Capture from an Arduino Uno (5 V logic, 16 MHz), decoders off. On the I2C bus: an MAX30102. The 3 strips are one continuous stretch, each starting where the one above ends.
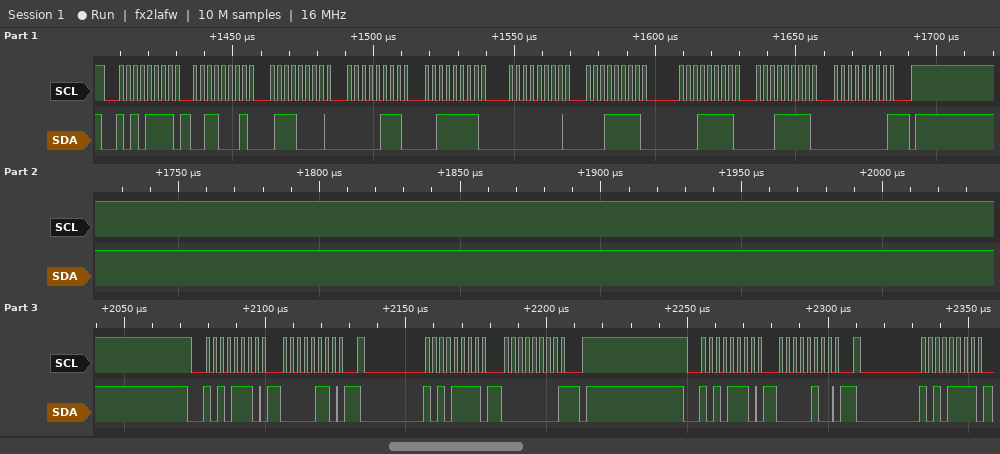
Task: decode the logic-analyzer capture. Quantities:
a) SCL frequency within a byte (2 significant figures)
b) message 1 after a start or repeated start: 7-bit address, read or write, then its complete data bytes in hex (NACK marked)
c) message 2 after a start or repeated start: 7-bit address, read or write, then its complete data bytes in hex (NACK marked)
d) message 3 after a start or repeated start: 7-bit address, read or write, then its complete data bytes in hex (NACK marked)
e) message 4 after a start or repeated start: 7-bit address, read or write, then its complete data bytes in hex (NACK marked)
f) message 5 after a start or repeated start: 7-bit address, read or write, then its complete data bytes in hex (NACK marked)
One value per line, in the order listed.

400 kHz
0x57 read: 31 70 07 3F 00 1F 1F 1F 00 NACK
0x57 write: 06
0x57 read: 00 NACK
0x57 write: 04
0x57 read
